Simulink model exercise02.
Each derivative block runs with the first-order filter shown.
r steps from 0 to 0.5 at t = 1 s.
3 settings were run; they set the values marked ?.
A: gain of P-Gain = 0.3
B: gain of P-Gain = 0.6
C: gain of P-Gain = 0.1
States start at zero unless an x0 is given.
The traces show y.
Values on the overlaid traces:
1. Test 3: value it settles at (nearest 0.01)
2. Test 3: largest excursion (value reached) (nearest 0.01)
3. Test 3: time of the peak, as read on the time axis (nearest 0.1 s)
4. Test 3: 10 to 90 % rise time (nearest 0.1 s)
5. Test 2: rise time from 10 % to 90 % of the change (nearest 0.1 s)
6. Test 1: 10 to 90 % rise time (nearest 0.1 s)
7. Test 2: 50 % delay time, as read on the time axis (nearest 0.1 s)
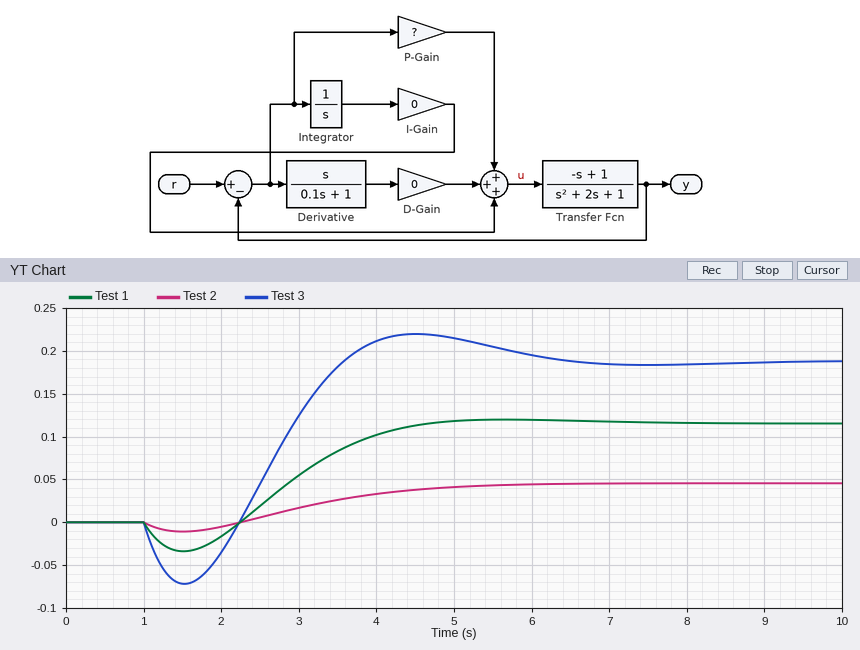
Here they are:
0.19
0.22
4.5 s
1.0 s
2.5 s
1.7 s
3.3 s
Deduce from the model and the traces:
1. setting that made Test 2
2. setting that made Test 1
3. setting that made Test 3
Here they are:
C
A
B
